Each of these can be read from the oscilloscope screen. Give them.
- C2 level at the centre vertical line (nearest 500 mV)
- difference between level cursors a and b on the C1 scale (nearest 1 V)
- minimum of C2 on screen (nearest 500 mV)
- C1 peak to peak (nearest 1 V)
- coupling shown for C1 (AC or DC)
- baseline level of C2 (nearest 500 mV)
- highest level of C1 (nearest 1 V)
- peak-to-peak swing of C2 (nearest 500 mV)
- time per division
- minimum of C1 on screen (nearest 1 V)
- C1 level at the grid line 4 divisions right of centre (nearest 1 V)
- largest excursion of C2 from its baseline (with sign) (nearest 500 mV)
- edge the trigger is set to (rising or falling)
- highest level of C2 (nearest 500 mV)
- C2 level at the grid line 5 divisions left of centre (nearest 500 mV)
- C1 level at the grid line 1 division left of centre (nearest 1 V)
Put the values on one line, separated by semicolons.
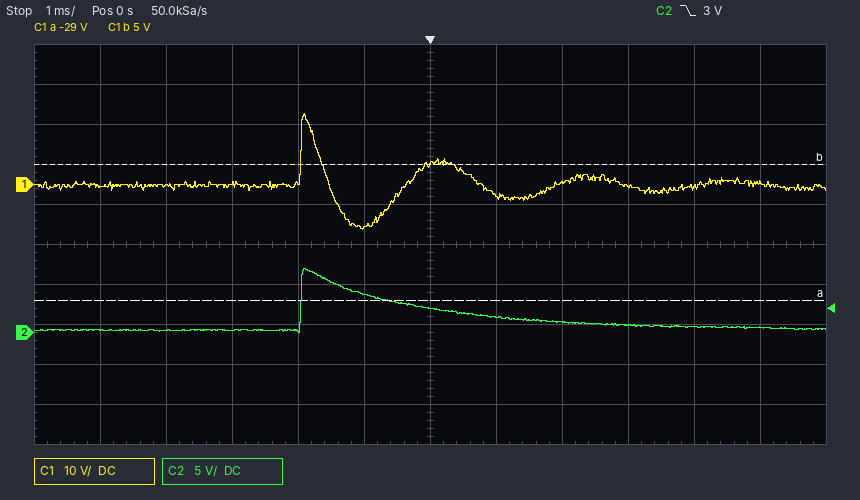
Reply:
3.0 V; 34 V; 0.0 V; 29 V; DC; 500 mV; 18 V; 8.0 V; 1 ms; -11 V; -1 V; +7.5 V; falling; 8.0 V; 500 mV; -11 V
